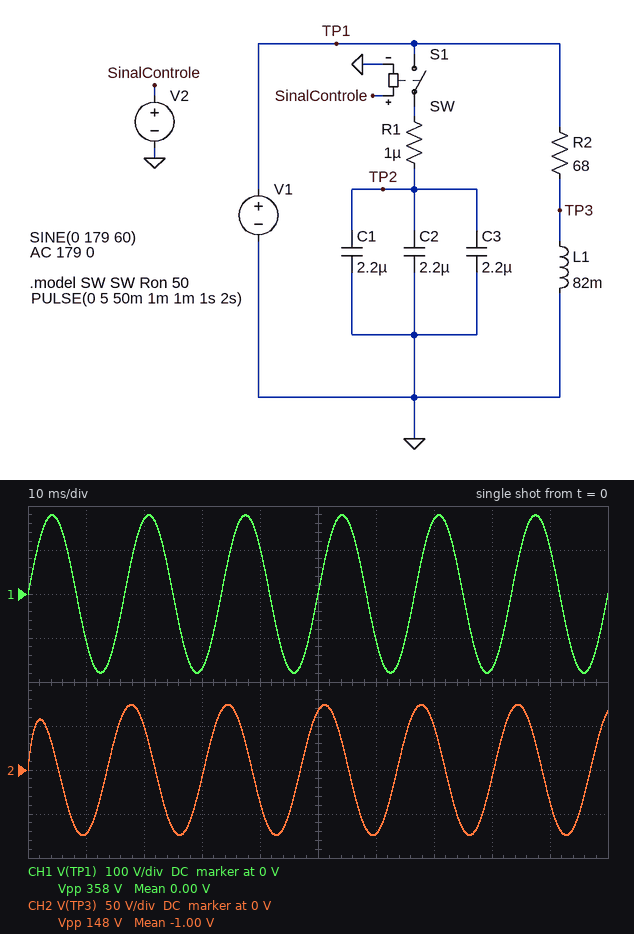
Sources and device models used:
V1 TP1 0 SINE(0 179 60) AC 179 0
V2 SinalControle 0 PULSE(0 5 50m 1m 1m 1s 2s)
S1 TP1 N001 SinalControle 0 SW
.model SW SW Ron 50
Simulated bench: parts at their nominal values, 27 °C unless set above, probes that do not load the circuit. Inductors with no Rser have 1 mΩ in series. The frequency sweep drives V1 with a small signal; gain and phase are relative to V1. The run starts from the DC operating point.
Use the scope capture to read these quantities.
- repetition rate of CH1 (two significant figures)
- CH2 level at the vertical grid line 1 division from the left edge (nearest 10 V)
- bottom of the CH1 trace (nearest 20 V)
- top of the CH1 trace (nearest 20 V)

60 Hz
-70 V
-180 V
180 V
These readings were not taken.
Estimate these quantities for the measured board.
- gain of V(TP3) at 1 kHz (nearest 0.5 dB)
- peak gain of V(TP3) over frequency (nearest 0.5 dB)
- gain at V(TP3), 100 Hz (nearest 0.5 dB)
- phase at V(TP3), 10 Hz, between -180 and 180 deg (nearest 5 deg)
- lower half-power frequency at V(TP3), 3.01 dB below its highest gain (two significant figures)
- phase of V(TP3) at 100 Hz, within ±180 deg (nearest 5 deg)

0 dB
0 dB
-4.5 dB
85 deg
130 Hz
55 deg
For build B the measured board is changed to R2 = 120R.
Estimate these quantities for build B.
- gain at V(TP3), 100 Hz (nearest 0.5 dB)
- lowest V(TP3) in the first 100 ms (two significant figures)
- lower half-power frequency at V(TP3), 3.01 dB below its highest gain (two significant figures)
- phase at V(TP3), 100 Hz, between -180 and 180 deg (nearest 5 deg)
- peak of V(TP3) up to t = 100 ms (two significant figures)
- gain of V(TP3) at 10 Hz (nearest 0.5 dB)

-8.0 dB
-45 V
230 Hz
65 deg
45 V
-27.5 dB
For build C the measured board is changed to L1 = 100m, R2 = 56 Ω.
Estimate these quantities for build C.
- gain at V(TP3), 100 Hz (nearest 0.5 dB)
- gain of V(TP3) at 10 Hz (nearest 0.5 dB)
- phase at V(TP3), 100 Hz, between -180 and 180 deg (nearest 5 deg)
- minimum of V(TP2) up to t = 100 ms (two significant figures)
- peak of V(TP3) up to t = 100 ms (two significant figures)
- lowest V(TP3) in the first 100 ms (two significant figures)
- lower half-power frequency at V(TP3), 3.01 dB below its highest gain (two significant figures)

-2.5 dB
-19.0 dB
40 deg
-180 V
100 V
-100 V
89 Hz
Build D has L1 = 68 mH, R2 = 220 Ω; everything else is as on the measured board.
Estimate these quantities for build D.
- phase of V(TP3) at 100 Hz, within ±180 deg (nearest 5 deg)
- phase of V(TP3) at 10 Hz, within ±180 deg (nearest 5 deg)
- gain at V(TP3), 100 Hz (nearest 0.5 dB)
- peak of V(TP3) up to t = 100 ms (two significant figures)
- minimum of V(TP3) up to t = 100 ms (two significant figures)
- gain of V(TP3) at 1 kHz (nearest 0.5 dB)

80 deg
90 deg
-14.5 dB
21 V
-21 V
-1.0 dB
